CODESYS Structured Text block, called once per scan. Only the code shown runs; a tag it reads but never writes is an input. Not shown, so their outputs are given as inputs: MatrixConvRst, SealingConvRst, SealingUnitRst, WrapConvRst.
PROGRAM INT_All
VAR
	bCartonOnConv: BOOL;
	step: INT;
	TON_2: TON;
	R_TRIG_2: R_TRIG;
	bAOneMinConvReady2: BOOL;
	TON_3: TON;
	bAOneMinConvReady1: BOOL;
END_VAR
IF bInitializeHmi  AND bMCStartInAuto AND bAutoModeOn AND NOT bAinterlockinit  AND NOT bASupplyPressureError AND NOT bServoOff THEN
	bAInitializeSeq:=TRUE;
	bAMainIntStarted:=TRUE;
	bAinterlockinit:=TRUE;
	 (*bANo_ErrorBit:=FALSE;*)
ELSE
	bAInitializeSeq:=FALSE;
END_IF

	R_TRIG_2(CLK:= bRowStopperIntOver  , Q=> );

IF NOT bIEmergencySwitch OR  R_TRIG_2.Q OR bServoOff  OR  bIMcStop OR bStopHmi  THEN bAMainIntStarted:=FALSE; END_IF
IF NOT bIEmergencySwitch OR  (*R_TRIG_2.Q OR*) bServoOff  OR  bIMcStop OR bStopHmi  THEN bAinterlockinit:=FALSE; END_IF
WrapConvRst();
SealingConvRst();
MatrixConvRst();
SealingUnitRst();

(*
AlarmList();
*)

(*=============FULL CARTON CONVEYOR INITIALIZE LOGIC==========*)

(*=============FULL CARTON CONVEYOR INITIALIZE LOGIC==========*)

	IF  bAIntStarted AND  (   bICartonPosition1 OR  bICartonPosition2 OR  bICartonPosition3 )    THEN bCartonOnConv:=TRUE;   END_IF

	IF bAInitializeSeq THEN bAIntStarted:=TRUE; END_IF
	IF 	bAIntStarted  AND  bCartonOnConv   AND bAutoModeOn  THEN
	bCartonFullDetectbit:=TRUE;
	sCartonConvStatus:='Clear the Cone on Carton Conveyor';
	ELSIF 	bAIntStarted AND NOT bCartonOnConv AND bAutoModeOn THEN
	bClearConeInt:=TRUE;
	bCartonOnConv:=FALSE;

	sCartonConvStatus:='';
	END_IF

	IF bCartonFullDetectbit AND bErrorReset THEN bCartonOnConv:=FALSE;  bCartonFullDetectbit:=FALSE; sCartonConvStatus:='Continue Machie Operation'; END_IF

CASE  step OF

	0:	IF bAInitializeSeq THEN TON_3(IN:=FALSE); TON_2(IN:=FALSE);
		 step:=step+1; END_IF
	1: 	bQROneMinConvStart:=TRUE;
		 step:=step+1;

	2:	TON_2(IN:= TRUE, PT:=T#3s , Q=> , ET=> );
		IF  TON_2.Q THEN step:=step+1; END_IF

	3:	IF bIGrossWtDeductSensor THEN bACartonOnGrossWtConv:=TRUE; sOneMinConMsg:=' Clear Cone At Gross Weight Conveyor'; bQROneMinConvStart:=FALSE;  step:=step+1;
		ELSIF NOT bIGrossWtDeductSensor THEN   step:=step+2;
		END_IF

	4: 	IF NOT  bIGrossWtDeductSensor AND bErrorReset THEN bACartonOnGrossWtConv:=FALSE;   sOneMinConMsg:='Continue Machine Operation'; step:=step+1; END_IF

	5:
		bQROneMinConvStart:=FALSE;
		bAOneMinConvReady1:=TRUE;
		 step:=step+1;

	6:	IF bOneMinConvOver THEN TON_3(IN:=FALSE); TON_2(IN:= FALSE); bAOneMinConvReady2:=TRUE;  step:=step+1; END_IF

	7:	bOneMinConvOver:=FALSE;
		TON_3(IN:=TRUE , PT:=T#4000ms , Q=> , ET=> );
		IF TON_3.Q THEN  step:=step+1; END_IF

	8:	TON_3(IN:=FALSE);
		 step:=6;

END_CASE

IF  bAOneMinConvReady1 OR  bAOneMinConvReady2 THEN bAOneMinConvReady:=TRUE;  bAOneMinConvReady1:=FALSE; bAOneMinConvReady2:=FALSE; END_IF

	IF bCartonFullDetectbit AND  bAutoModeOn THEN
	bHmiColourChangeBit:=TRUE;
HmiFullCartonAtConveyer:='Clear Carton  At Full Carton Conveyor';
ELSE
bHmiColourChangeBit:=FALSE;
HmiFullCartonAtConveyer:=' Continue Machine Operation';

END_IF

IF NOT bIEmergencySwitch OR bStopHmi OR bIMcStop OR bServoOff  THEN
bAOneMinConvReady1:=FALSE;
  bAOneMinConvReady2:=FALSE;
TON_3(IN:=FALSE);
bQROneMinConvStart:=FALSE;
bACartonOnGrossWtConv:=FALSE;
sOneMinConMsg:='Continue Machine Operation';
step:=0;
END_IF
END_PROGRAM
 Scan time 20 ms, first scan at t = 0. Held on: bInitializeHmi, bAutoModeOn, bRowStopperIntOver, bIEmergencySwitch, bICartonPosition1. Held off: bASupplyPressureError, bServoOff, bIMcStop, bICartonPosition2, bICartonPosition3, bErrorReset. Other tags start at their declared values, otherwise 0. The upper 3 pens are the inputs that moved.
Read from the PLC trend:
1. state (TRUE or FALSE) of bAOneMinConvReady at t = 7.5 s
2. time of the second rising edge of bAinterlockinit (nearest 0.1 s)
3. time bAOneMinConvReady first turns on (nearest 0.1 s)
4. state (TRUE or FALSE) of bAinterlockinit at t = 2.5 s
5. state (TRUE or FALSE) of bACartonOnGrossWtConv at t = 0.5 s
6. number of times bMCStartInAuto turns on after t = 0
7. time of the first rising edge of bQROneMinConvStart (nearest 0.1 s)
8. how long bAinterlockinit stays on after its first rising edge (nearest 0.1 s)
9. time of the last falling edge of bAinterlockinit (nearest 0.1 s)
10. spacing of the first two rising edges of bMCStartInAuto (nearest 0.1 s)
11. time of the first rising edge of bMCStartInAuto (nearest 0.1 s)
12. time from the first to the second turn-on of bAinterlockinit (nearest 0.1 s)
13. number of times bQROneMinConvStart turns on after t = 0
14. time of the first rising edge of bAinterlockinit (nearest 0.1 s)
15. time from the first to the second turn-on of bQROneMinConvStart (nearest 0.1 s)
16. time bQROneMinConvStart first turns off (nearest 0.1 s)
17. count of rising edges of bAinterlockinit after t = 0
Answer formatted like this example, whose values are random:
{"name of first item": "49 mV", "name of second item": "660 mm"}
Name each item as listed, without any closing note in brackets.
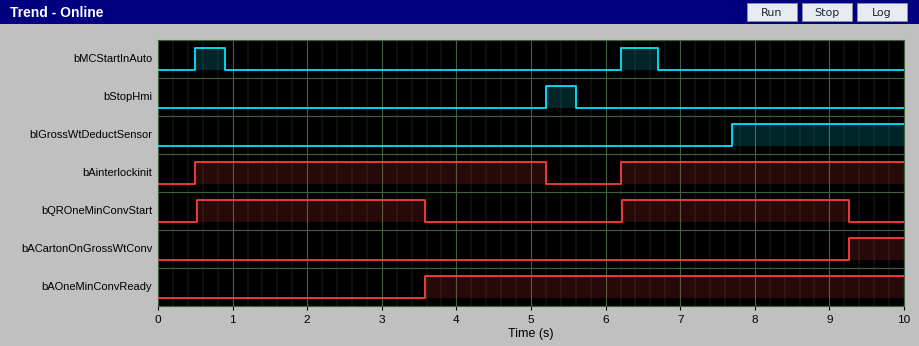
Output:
{"state (TRUE or FALSE) of bAOneMinConvReady at t = 7.5 s": "TRUE", "time of the second rising edge of bAinterlockinit": "6.2 s", "time bAOneMinConvReady first turns on": "3.6 s", "state (TRUE or FALSE) of bAinterlockinit at t = 2.5 s": "TRUE", "state (TRUE or FALSE) of bACartonOnGrossWtConv at t = 0.5 s": "FALSE", "number of times bMCStartInAuto turns on after t = 0": "2", "time of the first rising edge of bQROneMinConvStart": "0.5 s", "how long bAinterlockinit stays on after its first rising edge": "4.7 s", "time of the last falling edge of bAinterlockinit": "5.2 s", "spacing of the first two rising edges of bMCStartInAuto": "5.7 s", "time of the first rising edge of bMCStartInAuto": "0.5 s", "time from the first to the second turn-on of bAinterlockinit": "5.7 s", "number of times bQROneMinConvStart turns on after t = 0": "2", "time of the first rising edge of bAinterlockinit": "0.5 s", "time from the first to the second turn-on of bQROneMinConvStart": "5.7 s", "time bQROneMinConvStart first turns off": "3.6 s", "count of rising edges of bAinterlockinit after t = 0": "2"}
